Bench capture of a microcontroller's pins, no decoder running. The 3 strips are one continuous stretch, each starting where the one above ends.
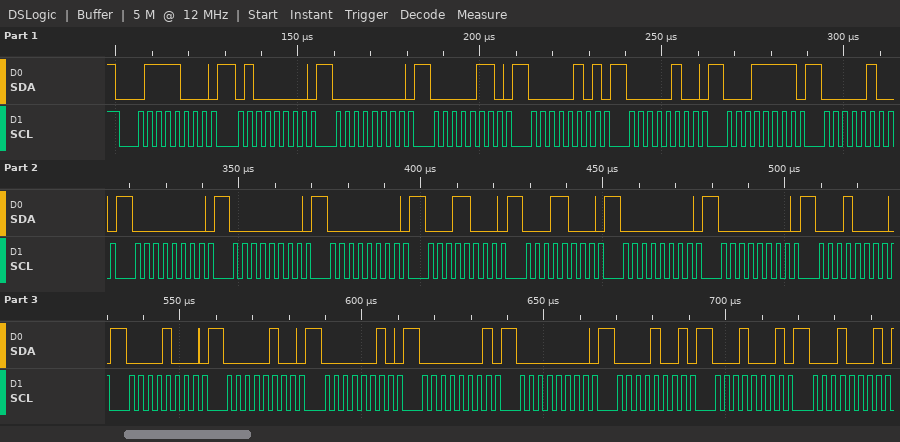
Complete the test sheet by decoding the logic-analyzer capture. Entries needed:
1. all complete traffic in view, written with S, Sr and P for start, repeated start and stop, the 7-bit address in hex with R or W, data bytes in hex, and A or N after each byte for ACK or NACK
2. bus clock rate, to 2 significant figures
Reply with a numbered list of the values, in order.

1. S 3CW A 40 A 00 A 06 A 05 A 04 A 1F A 04 A 00 A 00 A 00 A 18 A 18 A 00 A 00 A 10 A 08 A 04 A 02 A 01 A 00 A 09 A 11 A 11 A
2. 400 kHz
